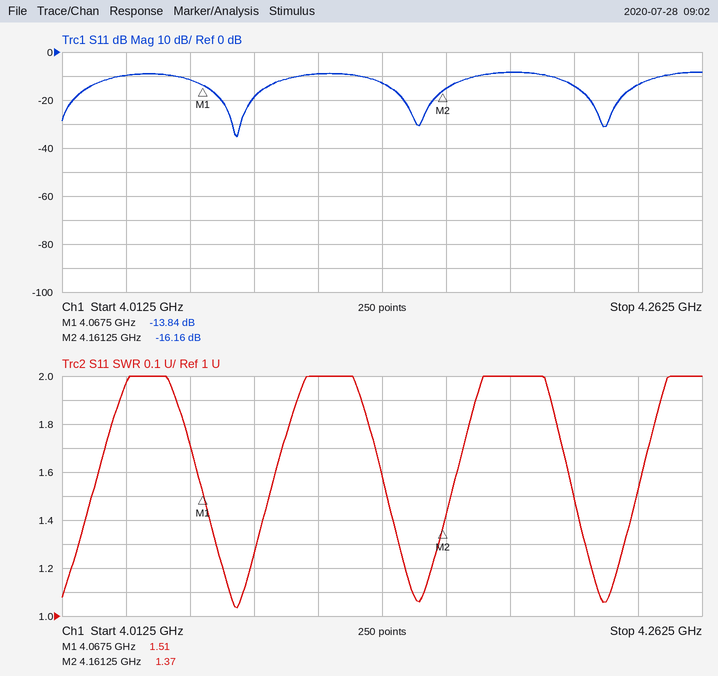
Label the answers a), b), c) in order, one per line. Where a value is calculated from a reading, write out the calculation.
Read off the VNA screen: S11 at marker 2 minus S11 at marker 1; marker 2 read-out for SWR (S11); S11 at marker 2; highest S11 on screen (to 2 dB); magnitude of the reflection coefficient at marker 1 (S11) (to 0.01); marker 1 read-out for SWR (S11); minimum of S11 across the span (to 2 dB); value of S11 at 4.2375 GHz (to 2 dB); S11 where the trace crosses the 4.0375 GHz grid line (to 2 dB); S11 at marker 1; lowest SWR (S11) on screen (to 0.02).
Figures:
a) -16.16 − (-13.84) = -2.32 dB
b) 1.37
c) -16.16 dB
d) -8 dB
e) 10^(-13.84/20) ≈ 0.20
f) 1.51
g) -36 dB
h) -14 dB
i) -10 dB
j) -13.84 dB
k) 1.04
